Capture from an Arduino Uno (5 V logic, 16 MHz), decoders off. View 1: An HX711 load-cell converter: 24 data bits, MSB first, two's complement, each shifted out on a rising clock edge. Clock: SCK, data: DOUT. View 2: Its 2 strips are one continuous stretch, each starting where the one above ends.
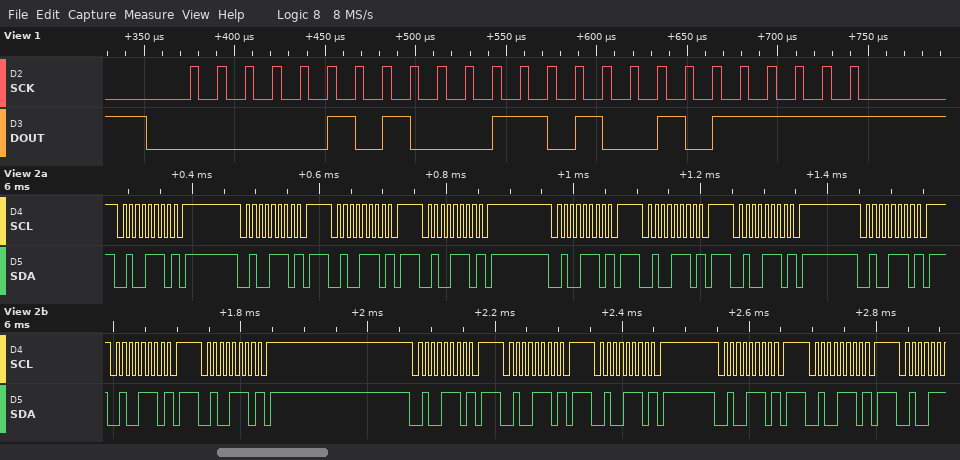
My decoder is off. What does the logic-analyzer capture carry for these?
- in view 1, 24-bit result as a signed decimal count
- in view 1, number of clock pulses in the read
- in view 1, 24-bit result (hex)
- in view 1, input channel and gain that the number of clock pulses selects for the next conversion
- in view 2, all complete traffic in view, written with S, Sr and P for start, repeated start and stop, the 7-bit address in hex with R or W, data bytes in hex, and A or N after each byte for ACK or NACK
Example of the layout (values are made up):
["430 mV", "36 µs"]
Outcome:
["334431", "25", "0x051A5F", "channel A, gain 128", "S 27W N P S 27W N P S 27W N P S 27W N P S 27W N P S 27W N P S 27W N P S 27W N P S 27W N P S 27W N P S 27W N P S 27W N P S 27W N P S 27W N P S 27W N P"]
